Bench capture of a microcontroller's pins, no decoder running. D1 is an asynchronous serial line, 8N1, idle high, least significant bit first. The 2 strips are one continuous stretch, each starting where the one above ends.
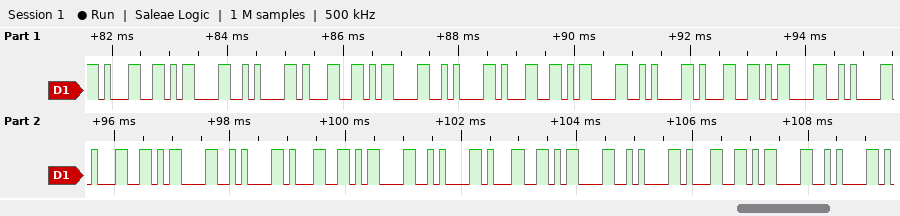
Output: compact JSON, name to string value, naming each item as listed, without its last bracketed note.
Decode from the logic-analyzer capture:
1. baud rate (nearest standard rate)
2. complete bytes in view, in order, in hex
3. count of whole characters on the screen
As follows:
{"baud rate": "9600 baud", "complete bytes in view, in order, in hex": "31 0D 0A 31 0D 0A 31 0D 0A 31 0D 0A 31 0D 0A 31 0D 0A 31 0D 0A 31 0D 0A", "count of whole characters on the screen": "24"}
